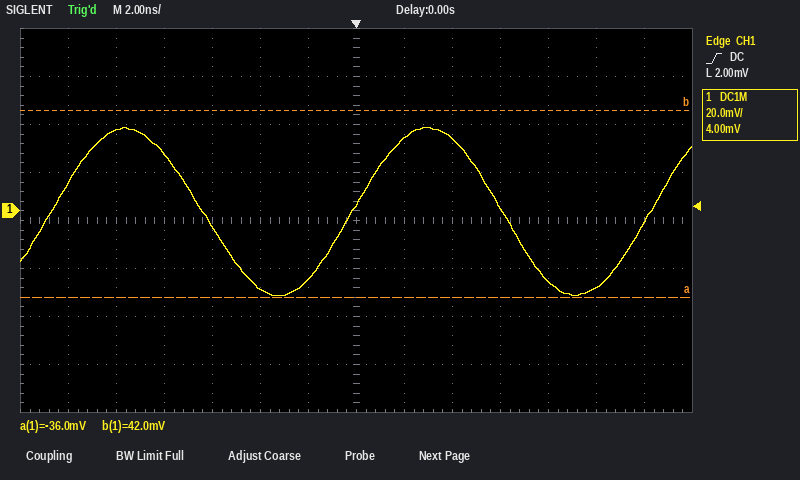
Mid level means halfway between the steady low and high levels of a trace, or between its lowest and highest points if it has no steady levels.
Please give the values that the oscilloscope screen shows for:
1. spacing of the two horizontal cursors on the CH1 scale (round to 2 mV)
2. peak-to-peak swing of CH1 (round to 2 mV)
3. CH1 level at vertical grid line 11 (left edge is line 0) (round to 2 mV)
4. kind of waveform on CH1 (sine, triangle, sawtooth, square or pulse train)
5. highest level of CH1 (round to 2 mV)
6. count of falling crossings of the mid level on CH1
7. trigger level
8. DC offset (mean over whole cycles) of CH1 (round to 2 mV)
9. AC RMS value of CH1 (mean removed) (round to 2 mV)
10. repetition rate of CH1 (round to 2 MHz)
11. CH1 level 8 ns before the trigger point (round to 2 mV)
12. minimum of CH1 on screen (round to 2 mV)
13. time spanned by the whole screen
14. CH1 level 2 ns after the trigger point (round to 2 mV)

78 mV
70 mV
-30 mV
sine
34 mV
2
2.00 mV
0 mV
24 mV
80 MHz
24 mV
-36 mV
28 ns
30 mV
